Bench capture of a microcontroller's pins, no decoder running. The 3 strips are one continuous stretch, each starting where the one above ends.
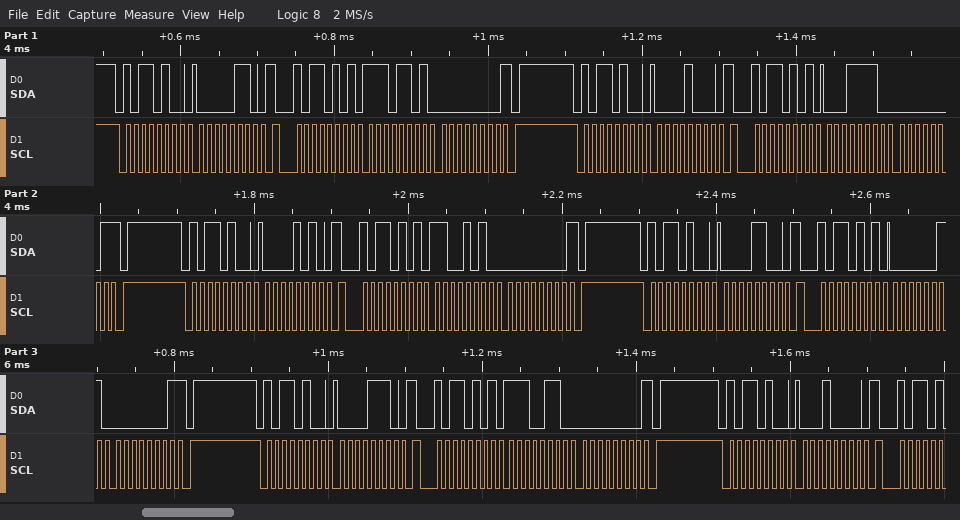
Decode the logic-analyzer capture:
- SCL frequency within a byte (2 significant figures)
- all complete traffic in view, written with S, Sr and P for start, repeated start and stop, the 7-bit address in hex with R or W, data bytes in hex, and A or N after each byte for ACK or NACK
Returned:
100 kHz
S 5AW A 06 A Sr 5AR A ED A 00 N P S 5AW A 08 A Sr 5AR A 1E A 01 N P S 5AW A 0A A Sr 5AR A CA A 00 N P S 5AW A 0C A Sr 5AR A 03 A 01 N P S 5AW A 0E A Sr 5AR A E6 A 00 N P S 5AW A 10 A
